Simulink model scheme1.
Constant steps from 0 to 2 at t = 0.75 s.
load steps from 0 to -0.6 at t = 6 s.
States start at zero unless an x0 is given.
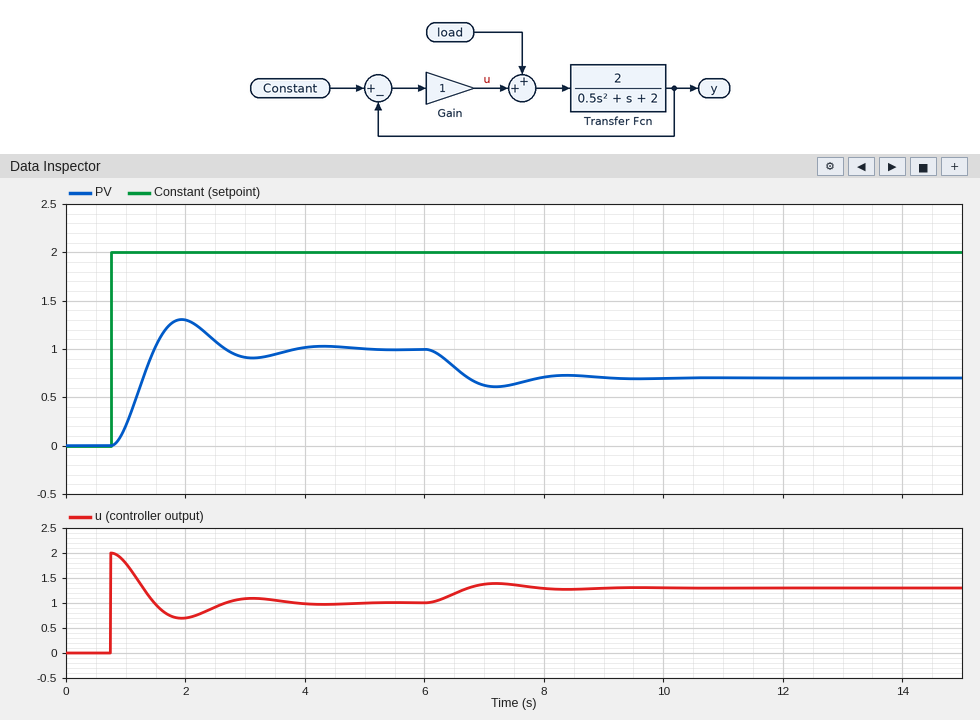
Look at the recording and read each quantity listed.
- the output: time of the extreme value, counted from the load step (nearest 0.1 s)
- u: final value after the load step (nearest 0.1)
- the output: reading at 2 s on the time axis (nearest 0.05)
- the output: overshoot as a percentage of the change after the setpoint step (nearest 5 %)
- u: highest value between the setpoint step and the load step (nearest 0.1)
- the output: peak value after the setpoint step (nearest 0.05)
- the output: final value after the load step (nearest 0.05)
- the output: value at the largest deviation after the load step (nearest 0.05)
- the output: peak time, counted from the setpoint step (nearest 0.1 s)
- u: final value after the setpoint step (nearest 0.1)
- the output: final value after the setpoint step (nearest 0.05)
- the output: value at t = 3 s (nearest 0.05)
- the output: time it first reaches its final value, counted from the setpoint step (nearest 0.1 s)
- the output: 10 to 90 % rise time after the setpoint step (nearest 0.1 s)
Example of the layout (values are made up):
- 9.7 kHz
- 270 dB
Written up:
- 1.2 s
- 1.3
- 1.30
- 30 %
- 2.0
- 1.30
- 0.70
- 0.60
- 1.2 s
- 1.0
- 1.00
- 0.90
- 0.7 s
- 0.5 s
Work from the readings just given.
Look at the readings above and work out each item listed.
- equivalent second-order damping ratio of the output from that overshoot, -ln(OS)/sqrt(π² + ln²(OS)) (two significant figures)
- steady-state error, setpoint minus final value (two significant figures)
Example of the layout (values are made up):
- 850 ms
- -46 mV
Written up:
- 0.36
- 1.0
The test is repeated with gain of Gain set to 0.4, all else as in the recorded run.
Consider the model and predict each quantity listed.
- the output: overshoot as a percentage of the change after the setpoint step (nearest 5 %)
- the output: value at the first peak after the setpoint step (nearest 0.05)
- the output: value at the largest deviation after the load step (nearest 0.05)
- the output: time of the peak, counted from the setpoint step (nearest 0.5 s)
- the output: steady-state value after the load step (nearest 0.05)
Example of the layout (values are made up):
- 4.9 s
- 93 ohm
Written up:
- 25 %
- 0.70
- 0.05
- 1.5 s
- 0.15
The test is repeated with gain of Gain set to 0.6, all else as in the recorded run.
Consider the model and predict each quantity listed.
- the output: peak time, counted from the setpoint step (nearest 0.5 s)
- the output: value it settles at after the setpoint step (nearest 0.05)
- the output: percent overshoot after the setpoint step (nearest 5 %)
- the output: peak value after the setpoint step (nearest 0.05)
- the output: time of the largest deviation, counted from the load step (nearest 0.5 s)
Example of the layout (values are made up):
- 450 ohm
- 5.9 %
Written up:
- 1.5 s
- 0.75
- 25 %
- 0.95
- 1.5 s
